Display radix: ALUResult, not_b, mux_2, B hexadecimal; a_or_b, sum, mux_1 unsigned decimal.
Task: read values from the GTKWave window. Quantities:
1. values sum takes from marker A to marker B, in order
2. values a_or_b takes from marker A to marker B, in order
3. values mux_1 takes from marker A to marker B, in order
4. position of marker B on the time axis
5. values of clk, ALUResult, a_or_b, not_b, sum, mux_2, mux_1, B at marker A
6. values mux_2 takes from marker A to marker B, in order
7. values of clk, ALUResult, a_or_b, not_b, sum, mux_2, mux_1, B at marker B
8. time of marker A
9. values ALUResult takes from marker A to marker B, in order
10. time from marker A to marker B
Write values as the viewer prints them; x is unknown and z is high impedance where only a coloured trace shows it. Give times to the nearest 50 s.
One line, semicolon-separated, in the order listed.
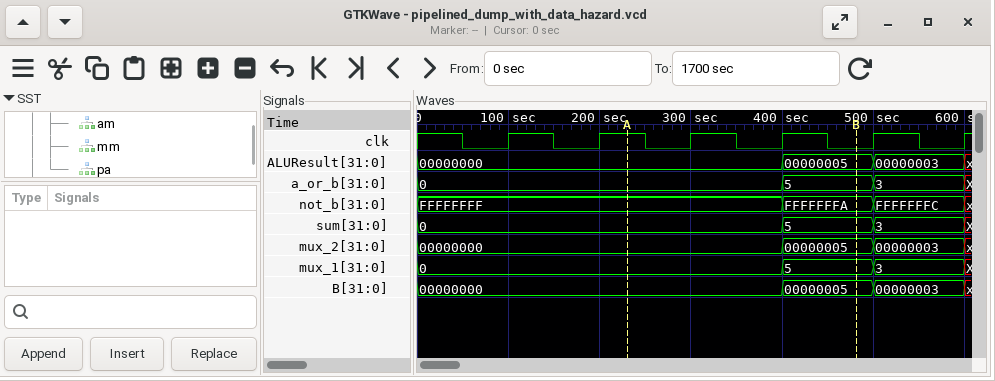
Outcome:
0, 5; 0, 5; 0, 5; 500 s; clk=1, ALUResult=00000000, a_or_b=0, not_b=FFFFFFFF, sum=0, mux_2=00000000, mux_1=0, B=00000000; 00000000, 00000005; clk=0, ALUResult=00000005, a_or_b=5, not_b=FFFFFFFA, sum=5, mux_2=00000005, mux_1=5, B=00000005; 250 s; 00000000, 00000005; 250 s
